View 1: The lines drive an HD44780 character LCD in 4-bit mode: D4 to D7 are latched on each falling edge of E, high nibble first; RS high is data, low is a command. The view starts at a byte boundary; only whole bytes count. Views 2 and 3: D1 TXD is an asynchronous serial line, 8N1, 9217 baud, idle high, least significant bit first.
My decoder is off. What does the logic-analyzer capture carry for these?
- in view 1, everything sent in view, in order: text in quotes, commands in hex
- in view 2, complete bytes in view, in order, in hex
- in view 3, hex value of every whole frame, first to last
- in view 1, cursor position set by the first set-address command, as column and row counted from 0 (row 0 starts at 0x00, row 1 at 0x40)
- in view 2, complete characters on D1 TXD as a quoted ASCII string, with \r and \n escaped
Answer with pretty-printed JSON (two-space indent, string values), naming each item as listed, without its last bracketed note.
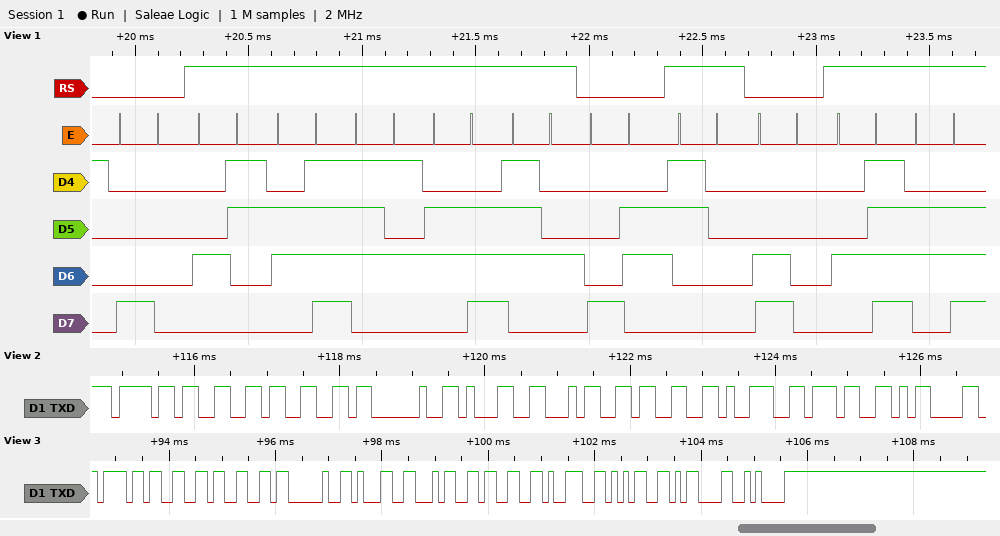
{
  "in view 1, everything sent in view, in order: text in quotes, commands in hex": "0x80 \"Count\" 0x86 \"0\" 0xC0 \"On\"",
  "in view 2, complete bytes in view, in order, in hex": "6F 66 66 20 31 34 33 39 37 0D",
  "in view 3, hex value of every whole frame, first to last": "6F 66 66 20 31 34 33 39 35 0D 0A",
  "in view 1, cursor position set by the first set-address command, as column and row counted from 0": "column 0, row 0",
  "in view 2, complete characters on D1 TXD as a quoted ASCII string, with \\r and \\n escaped": "\"off 14397\\r\""
}
